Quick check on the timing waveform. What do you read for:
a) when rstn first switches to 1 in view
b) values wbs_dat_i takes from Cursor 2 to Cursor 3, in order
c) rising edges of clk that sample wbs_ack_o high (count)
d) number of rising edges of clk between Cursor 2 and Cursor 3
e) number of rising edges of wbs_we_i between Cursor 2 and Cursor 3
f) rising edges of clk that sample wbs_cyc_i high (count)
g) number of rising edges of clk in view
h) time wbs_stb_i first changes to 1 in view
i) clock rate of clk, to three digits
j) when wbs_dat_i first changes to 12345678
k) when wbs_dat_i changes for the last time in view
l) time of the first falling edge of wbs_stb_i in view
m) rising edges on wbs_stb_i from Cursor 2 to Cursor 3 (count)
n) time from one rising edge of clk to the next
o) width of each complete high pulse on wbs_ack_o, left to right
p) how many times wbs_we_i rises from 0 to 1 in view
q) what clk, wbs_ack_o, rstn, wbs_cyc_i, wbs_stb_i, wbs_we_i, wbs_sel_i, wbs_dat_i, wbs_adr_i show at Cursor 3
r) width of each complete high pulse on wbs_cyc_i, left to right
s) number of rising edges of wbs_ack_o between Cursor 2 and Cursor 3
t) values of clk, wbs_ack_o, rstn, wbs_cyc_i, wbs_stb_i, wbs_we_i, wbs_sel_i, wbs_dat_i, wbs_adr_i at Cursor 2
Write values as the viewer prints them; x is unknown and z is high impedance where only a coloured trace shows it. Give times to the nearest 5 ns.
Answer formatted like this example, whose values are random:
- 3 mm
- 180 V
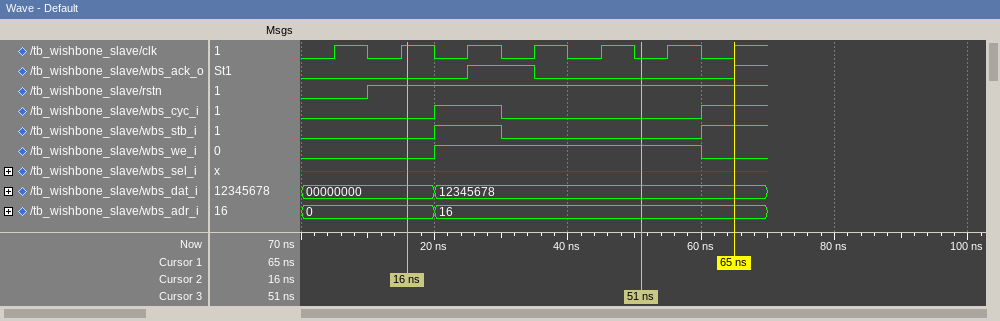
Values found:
- 10 ns
- 00000000, 12345678
- 1
- 3
- 1
- 2
- 7
- 20 ns
- 100 MHz
- 20 ns
- 20 ns
- 30 ns
- 1
- 10 ns
- 10 ns
- 1
- clk=0, wbs_ack_o=0, rstn=1, wbs_cyc_i=0, wbs_stb_i=0, wbs_we_i=1, wbs_sel_i=x, wbs_dat_i=12345678, wbs_adr_i=16
- 10 ns
- 1
- clk=1, wbs_ack_o=0, rstn=1, wbs_cyc_i=0, wbs_stb_i=0, wbs_we_i=0, wbs_sel_i=x, wbs_dat_i=00000000, wbs_adr_i=0
